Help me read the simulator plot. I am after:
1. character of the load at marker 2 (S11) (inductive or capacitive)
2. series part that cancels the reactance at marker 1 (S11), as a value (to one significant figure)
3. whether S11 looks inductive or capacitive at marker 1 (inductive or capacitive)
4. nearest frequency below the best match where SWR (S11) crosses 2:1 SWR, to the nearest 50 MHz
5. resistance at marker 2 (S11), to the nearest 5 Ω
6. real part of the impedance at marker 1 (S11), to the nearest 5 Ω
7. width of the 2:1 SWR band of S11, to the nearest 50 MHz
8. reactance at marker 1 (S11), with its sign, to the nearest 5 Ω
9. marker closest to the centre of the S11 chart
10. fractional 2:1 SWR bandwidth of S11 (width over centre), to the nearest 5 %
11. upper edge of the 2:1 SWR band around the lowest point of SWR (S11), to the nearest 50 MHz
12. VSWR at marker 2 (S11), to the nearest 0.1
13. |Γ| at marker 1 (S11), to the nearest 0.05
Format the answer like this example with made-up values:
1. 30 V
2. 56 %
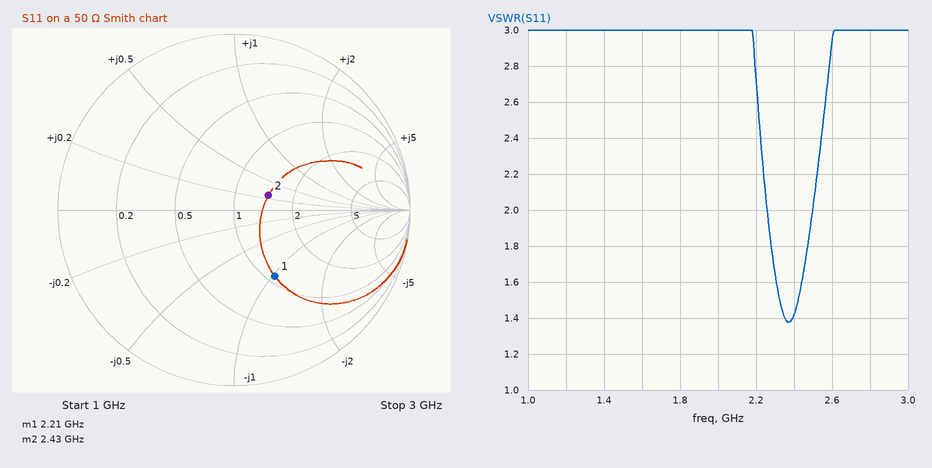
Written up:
1. inductive
2. 4 nH
3. capacitive
4. 2.25 GHz
5. 75 Ω
6. 55 Ω
7. 250 MHz
8. -50 Ω
9. marker 2
10. 10 %
11. 2.50 GHz
12. 1.5
13. 0.45
